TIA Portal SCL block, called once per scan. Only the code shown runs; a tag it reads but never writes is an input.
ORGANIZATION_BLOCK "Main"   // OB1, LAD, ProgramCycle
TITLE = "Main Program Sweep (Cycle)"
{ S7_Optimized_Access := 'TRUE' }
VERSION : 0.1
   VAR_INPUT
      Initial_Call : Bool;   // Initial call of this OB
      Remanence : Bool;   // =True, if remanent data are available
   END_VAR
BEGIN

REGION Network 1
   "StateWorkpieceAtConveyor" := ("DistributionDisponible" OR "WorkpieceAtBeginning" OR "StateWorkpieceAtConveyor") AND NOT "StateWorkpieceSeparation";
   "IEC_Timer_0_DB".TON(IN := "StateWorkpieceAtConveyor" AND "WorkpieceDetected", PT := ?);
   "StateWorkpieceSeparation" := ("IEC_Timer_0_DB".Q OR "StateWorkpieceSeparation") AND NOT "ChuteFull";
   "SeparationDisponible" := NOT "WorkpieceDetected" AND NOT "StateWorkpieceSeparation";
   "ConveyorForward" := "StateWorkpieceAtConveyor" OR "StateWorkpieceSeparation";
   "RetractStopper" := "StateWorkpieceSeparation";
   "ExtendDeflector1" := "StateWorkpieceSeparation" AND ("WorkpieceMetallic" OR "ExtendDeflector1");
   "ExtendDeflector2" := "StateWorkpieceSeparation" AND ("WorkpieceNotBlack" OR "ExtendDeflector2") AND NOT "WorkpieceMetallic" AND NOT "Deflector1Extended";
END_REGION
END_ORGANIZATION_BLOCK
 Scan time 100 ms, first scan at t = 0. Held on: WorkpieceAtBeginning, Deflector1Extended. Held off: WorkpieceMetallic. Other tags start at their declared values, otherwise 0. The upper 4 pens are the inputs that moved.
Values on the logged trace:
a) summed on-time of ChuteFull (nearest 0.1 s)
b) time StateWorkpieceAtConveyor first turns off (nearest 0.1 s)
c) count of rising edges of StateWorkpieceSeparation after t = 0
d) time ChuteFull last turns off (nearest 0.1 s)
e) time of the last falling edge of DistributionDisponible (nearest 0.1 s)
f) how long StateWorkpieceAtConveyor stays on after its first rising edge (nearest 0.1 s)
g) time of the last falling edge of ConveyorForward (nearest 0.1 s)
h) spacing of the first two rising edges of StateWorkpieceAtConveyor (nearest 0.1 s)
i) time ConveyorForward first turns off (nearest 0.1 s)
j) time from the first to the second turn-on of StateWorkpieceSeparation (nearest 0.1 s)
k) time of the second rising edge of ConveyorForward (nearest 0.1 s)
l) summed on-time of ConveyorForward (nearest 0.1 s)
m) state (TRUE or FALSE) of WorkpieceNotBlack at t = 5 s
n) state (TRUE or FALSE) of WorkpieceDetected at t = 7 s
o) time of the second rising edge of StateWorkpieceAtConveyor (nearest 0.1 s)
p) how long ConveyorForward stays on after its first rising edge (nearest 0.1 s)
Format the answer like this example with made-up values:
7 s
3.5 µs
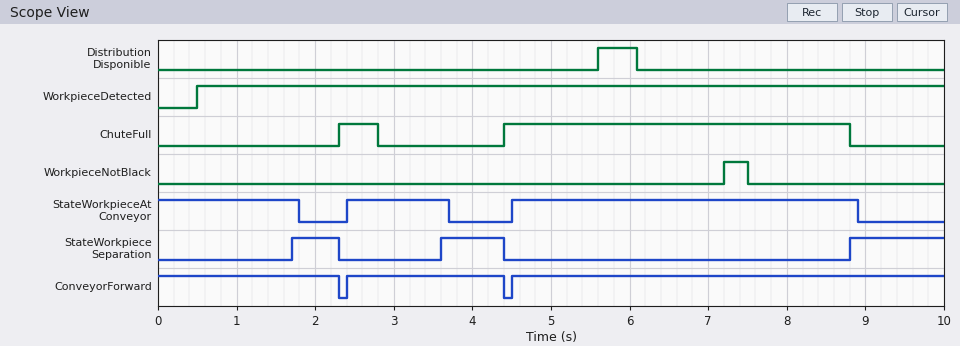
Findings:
4.9 s
1.8 s
3
8.8 s
6.1 s
1.3 s
4.4 s
2.1 s
2.3 s
1.9 s
4.5 s
9.8 s
FALSE
TRUE
4.5 s
2.0 s
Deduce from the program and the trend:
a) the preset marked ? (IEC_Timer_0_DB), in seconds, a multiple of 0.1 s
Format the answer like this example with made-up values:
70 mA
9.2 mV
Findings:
1.2 s
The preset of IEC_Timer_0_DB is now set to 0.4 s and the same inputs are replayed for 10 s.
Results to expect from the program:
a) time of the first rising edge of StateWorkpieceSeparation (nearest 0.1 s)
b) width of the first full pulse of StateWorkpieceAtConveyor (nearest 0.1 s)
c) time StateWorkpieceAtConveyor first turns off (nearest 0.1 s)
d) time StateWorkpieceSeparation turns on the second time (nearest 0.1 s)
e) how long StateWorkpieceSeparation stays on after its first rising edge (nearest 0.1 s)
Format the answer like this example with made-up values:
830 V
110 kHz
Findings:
0.9 s
0.5 s
1.0 s
2.8 s
1.4 s
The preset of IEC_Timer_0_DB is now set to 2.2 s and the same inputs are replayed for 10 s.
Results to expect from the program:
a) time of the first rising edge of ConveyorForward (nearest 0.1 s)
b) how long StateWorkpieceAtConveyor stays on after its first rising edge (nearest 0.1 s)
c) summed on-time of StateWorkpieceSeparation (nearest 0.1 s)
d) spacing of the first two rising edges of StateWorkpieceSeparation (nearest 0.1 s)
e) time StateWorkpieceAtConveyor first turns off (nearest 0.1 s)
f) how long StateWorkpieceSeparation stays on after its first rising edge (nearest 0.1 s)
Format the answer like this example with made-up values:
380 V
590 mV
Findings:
4.5 s
4.4 s
2.8 s
6.0 s
2.9 s
1.6 s
